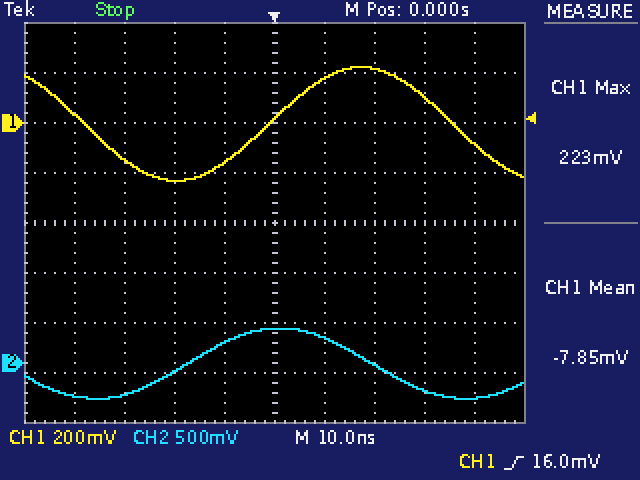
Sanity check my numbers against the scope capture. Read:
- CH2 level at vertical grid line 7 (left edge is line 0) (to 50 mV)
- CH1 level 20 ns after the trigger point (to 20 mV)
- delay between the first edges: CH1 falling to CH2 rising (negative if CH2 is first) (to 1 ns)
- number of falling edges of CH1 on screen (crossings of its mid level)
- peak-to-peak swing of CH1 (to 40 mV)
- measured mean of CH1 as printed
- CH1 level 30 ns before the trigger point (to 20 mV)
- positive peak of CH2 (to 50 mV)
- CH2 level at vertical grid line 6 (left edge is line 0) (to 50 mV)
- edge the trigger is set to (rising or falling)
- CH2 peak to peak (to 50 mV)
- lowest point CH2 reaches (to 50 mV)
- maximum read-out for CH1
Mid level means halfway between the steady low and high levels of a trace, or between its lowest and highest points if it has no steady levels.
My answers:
0 mV
220 mV
+21 ns
2
440 mV
-7.85 mV
-140 mV
350 mV
250 mV
rising
700 mV
-350 mV
223 mV
